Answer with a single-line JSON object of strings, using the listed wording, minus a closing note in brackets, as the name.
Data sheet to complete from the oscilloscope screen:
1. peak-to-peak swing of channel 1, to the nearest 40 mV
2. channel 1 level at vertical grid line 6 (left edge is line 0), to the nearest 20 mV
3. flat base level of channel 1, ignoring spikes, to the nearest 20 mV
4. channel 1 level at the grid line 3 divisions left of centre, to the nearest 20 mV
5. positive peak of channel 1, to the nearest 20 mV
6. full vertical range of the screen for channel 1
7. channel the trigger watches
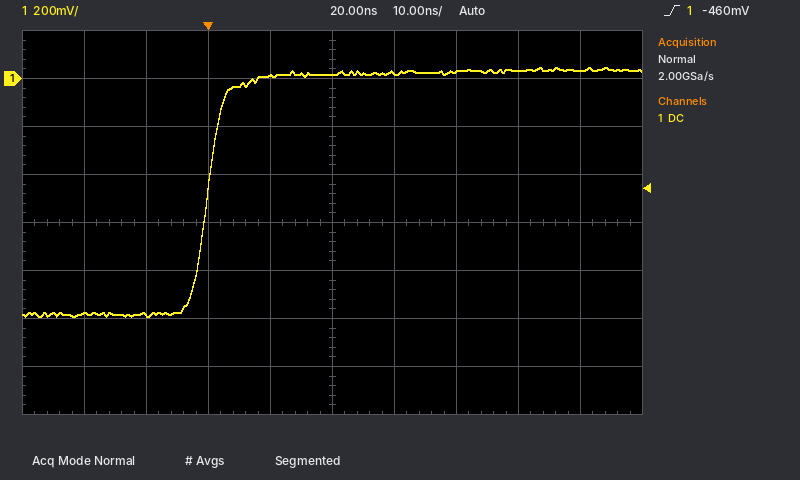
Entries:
{"peak-to-peak swing of channel 1, to the nearest 40 mV": "1.04 V", "channel 1 level at vertical grid line 6 (left edge is line 0), to the nearest 20 mV": "20 mV", "flat base level of channel 1, ignoring spikes, to the nearest 20 mV": "-980 mV", "channel 1 level at the grid line 3 divisions left of centre, to the nearest 20 mV": "-980 mV", "positive peak of channel 1, to the nearest 20 mV": "40 mV", "full vertical range of the screen for channel 1": "1.6 V", "channel the trigger watches": "channel 1"}
